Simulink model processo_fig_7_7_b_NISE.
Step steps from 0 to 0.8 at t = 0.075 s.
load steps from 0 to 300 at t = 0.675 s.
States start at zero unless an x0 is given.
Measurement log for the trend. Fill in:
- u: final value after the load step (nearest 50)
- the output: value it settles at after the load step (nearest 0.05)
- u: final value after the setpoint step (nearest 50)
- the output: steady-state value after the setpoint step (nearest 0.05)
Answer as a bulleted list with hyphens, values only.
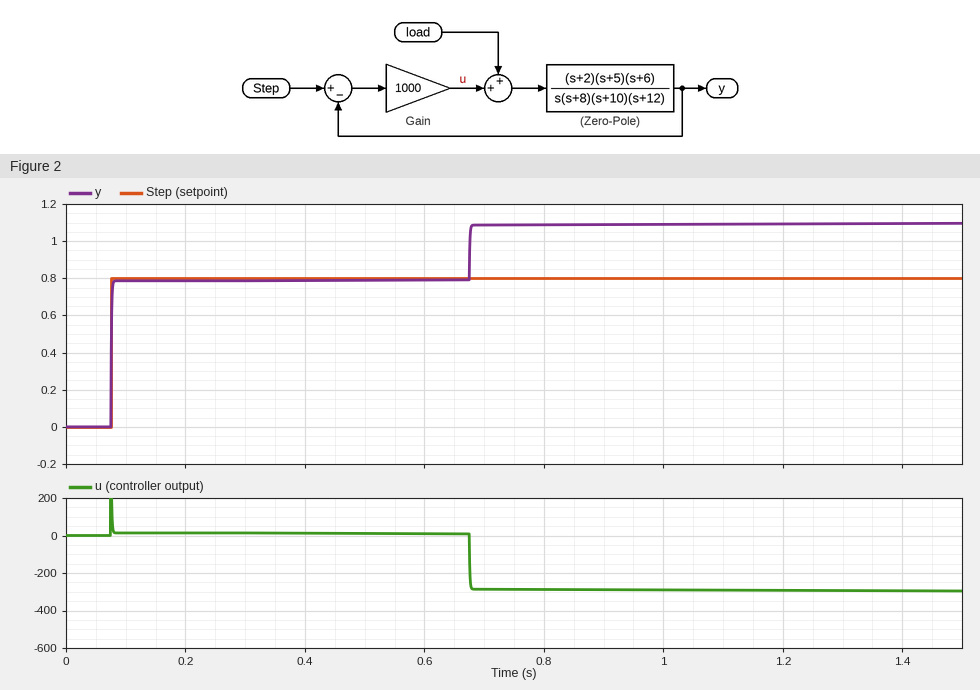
- -300
- 1.10
- 0
- 0.80
